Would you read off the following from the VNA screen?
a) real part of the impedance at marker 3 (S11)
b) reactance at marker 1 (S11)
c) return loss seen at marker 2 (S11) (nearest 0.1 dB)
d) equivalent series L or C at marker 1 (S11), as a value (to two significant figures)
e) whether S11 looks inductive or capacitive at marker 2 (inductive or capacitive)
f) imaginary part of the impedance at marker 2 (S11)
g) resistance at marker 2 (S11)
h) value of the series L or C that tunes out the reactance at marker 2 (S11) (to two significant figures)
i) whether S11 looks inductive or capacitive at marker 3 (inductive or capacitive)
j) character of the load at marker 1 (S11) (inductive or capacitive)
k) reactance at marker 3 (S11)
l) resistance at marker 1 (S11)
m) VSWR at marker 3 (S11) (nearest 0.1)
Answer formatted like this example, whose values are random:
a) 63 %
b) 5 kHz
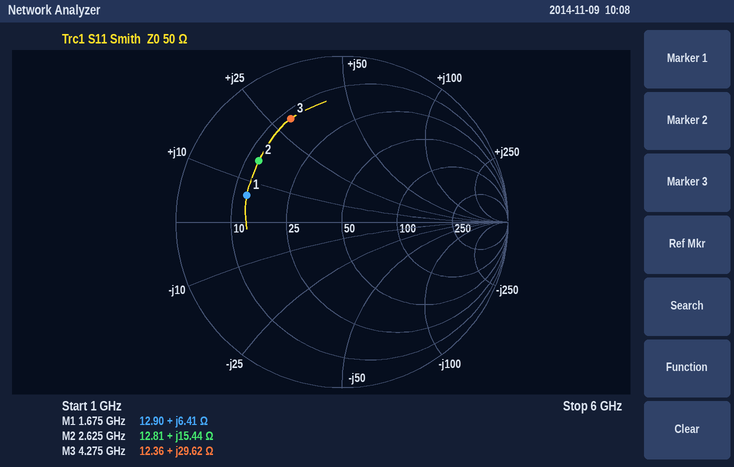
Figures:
a) 12.36 Ω
b) +6.41 Ω
c) 4.1 dB
d) 610 pH
e) inductive
f) +15.44 Ω
g) 12.81 Ω
h) 3.9 pF
i) inductive
j) inductive
k) +29.62 Ω
l) 12.90 Ω
m) 5.5
